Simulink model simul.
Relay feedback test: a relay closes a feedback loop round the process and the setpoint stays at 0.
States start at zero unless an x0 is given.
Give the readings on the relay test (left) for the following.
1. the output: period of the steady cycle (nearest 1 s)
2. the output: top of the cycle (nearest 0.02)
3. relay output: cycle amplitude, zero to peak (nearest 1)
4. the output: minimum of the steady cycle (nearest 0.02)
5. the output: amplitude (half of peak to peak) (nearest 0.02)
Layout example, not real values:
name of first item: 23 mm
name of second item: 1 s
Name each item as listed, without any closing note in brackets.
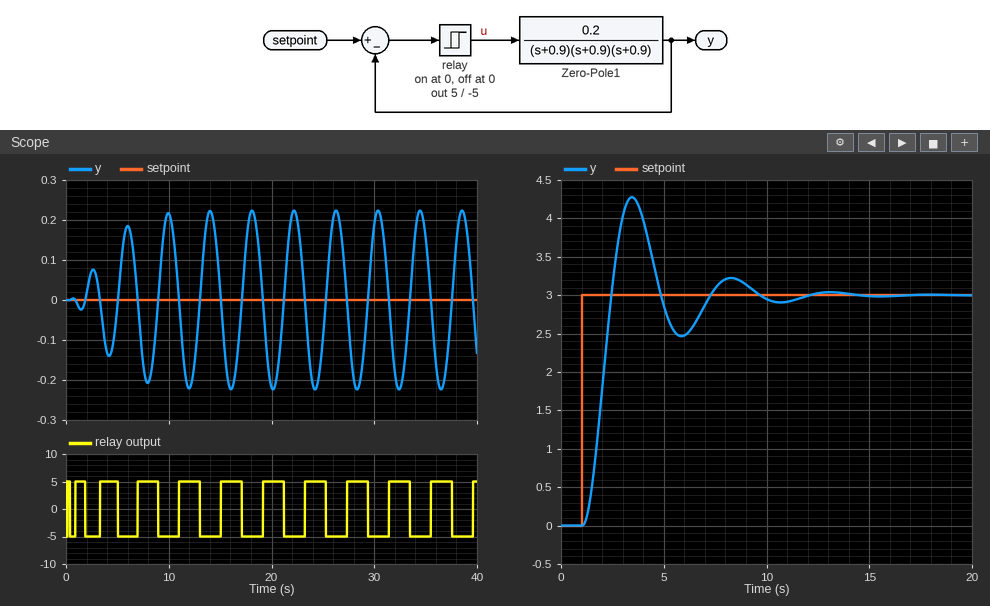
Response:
the output: period of the steady cycle: 4 s
the output: top of the cycle: 0.22
relay output: cycle amplitude, zero to peak: 5
the output: minimum of the steady cycle: -0.22
the output: amplitude (half of peak to peak): 0.22
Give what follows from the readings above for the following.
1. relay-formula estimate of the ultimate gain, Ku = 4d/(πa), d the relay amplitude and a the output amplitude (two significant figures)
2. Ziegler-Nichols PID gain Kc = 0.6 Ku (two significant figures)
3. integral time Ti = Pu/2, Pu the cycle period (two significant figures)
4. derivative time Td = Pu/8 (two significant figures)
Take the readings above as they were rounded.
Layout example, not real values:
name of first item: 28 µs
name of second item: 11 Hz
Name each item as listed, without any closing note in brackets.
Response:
relay-formula estimate of the ultimate gain, Ku = 4d/(πa), d the relay amplitude and a the output amplitude: 29
Ziegler-Nichols PID gain Kc = 0.6 Ku: 17
integral time Ti = Pu/2, Pu the cycle period: 2.0 s
derivative time Td = Pu/8: 0.50 s
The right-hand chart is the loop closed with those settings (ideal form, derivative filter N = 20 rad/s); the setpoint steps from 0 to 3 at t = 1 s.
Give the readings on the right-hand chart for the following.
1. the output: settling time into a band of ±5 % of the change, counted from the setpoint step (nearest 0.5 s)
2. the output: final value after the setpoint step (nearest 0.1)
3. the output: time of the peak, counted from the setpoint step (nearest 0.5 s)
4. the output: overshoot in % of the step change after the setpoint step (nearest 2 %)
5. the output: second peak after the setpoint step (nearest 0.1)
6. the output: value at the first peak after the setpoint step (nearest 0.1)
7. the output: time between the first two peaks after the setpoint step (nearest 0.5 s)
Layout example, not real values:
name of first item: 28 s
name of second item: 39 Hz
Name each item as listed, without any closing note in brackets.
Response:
the output: settling time into a band of ±5 % of the change, counted from the setpoint step: 8.0 s
the output: final value after the setpoint step: 3.0
the output: time of the peak, counted from the setpoint step: 2.5 s
the output: overshoot in % of the step change after the setpoint step: 42 %
the output: second peak after the setpoint step: 3.2
the output: value at the first peak after the setpoint step: 4.3
the output: time between the first two peaks after the setpoint step: 5.0 s
